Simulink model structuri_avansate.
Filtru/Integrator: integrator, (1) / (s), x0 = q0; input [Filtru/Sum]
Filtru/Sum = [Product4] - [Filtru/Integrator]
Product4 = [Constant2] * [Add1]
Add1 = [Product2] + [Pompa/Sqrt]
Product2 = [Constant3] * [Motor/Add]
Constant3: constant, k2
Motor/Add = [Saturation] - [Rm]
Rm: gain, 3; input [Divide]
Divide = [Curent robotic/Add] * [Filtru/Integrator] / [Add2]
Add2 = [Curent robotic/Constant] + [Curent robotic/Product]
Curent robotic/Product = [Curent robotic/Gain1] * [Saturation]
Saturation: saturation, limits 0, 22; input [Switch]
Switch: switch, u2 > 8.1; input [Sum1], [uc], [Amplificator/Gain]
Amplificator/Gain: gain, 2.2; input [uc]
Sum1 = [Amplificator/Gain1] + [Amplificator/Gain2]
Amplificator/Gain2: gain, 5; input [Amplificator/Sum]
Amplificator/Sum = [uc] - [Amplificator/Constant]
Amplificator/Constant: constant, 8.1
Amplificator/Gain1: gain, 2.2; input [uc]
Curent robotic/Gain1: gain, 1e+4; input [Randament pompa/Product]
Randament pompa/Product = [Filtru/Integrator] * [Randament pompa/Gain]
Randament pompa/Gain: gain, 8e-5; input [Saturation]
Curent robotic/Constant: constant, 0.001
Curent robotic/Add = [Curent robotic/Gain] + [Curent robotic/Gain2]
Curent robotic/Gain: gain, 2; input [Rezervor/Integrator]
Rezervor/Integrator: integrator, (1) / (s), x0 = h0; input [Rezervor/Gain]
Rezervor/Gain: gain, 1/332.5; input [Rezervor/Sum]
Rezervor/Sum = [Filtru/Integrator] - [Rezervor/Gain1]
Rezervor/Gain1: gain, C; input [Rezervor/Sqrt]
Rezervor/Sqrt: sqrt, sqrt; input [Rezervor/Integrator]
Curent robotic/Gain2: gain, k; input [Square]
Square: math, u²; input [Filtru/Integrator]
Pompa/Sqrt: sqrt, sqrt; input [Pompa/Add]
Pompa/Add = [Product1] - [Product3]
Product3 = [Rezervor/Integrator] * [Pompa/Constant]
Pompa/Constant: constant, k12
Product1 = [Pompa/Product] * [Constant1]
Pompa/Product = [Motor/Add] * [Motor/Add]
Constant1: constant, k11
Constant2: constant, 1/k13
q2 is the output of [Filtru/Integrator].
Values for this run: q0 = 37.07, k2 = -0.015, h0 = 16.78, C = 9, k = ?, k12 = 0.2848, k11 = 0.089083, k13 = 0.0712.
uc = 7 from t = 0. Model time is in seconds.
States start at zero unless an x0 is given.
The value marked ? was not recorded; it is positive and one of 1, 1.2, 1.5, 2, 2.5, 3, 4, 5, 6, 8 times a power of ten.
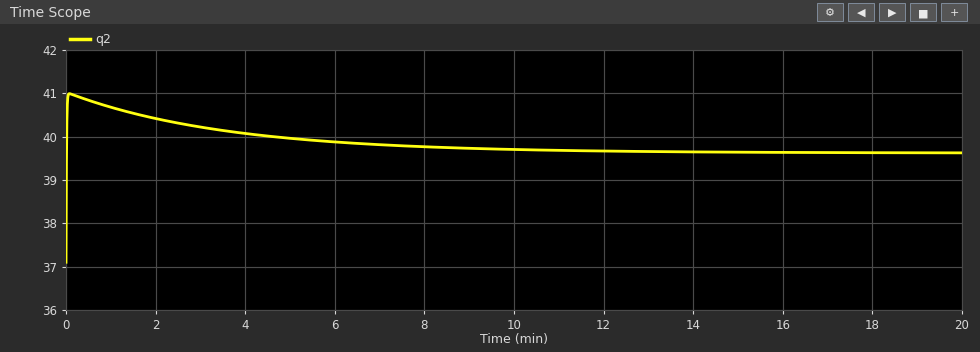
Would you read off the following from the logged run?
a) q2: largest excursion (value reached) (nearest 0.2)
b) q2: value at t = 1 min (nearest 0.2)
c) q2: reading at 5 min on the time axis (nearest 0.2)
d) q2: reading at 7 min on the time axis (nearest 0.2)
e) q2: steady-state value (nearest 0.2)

41.0
40.6
40.0
39.8
39.6
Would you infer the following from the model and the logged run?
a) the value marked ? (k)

0.08
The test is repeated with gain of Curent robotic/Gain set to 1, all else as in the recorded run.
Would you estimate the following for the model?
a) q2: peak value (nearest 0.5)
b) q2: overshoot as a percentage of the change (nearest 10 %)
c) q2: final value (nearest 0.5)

42.0
50 %
40.5
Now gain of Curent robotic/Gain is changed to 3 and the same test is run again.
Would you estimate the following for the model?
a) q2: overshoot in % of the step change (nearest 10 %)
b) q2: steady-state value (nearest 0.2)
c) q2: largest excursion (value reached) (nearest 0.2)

60 %
39.0
40.2
